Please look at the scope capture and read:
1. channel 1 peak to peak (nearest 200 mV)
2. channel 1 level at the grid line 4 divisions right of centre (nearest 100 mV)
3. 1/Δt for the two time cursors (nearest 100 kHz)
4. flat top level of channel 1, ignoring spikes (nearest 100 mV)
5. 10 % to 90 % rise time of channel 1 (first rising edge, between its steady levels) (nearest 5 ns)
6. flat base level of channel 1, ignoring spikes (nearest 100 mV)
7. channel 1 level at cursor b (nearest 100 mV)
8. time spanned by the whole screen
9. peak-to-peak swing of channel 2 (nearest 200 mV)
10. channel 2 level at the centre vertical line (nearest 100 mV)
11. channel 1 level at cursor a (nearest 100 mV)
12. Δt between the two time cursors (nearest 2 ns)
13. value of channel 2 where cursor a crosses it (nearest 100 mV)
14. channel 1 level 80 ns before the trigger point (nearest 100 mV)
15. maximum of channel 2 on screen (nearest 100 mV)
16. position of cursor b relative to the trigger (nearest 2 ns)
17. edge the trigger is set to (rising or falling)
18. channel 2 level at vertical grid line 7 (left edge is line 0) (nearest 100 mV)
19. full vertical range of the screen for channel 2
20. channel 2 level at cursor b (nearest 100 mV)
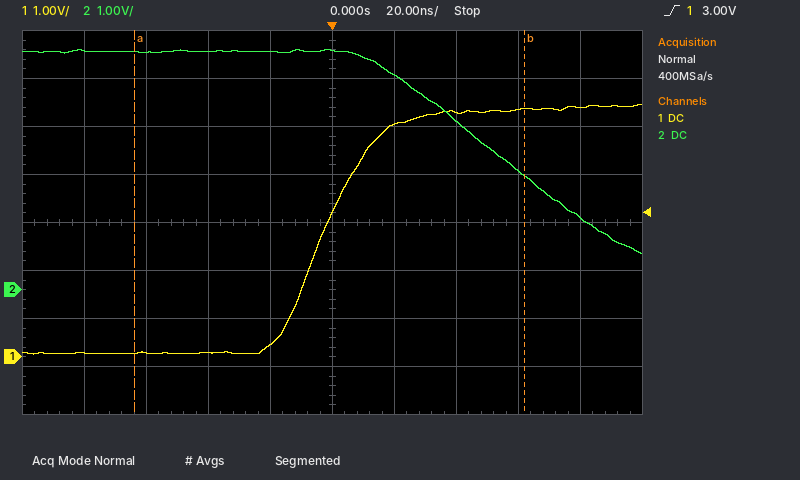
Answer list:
5.2 V
5.2 V
7.9 MHz
5.2 V
30 ns
100 mV
5.2 V
200 ns
4.2 V
5.0 V
100 mV
126 ns
5.0 V
100 mV
5.0 V
+62 ns
rising
3.5 V
8 V
2.4 V
